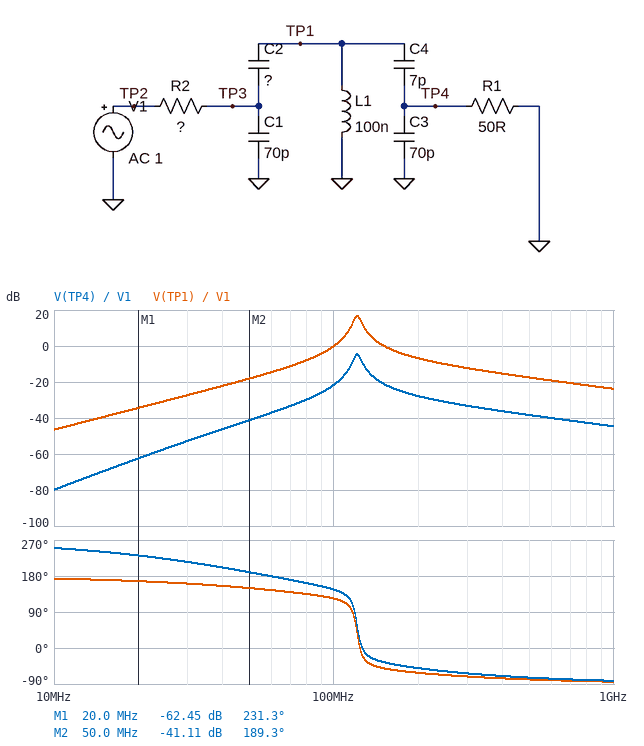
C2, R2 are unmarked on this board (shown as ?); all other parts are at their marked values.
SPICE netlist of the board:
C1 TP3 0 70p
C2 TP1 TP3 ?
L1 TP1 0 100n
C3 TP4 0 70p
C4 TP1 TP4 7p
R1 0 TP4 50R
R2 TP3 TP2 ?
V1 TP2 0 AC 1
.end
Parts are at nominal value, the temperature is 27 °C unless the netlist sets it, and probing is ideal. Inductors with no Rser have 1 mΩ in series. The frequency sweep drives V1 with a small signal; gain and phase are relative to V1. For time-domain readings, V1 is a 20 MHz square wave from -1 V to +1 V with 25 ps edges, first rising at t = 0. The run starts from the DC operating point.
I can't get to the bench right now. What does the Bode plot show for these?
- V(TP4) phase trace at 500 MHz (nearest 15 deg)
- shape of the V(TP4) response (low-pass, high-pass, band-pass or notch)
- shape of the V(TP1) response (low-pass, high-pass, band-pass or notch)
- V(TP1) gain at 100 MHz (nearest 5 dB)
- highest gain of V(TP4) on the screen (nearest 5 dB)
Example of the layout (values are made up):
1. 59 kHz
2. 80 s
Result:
1. -75 deg
2. band-pass
3. band-pass
4. 0 dB
5. -5 dB
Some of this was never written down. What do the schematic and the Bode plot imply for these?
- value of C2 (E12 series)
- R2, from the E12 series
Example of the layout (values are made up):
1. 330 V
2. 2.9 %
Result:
1. 12 pF
2. 22 Ω
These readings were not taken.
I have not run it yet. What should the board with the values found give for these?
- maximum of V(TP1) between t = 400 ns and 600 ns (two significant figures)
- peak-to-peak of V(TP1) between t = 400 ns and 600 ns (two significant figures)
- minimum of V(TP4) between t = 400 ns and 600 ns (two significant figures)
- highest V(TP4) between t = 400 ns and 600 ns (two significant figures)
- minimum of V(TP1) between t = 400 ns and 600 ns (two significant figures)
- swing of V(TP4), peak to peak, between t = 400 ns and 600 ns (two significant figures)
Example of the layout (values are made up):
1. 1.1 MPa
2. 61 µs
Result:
1. 510 mV
2. 1.0 V
3. -41 mV
4. 41 mV
5. -510 mV
6. 81 mV
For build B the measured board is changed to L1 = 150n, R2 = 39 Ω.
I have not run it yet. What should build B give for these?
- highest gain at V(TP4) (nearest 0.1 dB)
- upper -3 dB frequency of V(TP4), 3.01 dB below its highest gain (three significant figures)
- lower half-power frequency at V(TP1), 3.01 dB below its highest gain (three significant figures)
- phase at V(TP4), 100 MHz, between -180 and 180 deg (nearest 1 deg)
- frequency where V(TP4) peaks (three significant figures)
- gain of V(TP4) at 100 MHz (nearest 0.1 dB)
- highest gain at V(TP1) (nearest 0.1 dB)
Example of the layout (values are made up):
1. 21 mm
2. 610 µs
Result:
1. -6.3 dB
2. 102 MHz
3. 96.8 MHz
4. 39 deg
5. 99.5 MHz
6. -6.4 dB
7. 15.2 dB
